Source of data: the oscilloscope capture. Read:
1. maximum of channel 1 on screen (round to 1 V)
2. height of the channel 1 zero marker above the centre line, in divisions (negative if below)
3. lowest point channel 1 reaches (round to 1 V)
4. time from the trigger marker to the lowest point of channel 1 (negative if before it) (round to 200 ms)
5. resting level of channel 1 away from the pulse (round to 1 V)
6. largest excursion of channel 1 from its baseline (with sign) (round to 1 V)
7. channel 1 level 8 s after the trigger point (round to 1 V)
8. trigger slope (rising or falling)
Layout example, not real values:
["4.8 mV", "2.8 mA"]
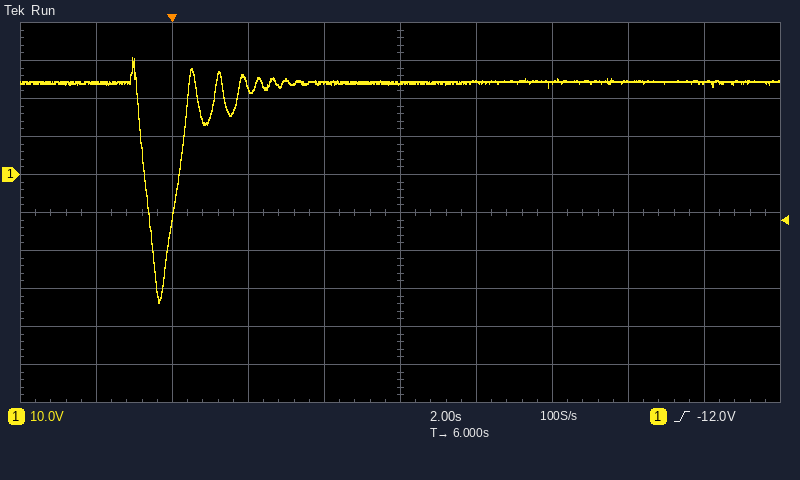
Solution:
["31 V", "+1.0 div", "-34 V", "-400 ms", "24 V", "-58 V", "24 V", "rising"]
